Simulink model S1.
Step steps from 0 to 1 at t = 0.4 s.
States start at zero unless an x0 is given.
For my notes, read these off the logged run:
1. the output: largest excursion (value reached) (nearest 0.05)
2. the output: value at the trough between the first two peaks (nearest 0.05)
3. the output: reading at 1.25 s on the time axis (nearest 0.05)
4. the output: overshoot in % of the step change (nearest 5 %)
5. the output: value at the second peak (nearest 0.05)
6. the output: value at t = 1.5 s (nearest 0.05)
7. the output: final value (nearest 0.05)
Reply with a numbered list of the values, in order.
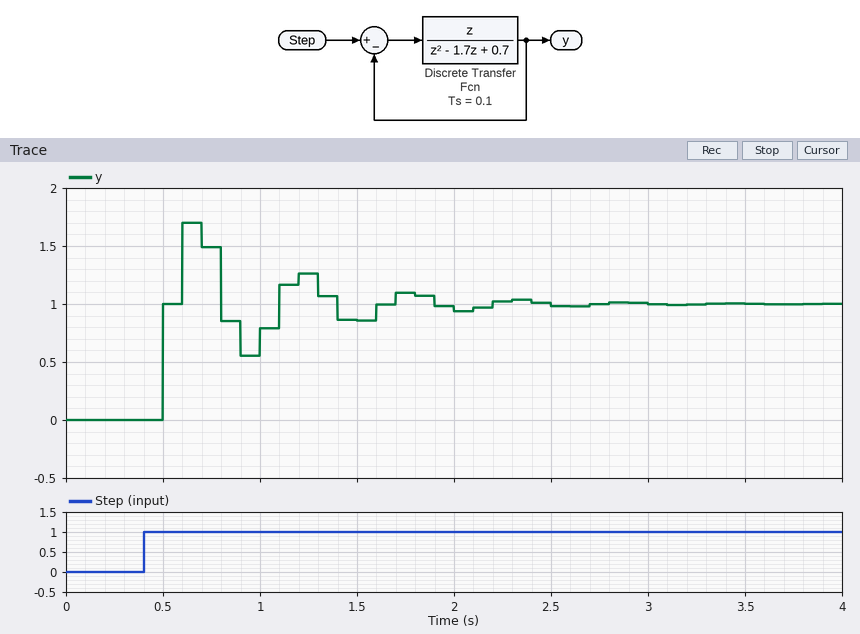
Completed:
1. 1.70
2. 0.55
3. 1.25
4. 70 %
5. 1.25
6. 0.85
7. 1.00
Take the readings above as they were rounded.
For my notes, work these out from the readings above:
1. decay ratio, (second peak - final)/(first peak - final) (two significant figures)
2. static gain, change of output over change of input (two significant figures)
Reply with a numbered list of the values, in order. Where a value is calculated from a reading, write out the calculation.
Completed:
1. (1.25 - 1) / (1.7 - 1) = 0.36
2. (1 - 0) / (1 - 0) = 1.0
